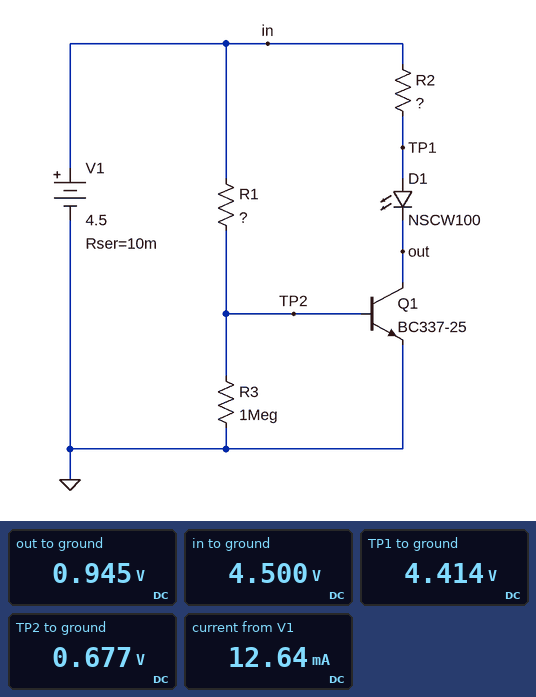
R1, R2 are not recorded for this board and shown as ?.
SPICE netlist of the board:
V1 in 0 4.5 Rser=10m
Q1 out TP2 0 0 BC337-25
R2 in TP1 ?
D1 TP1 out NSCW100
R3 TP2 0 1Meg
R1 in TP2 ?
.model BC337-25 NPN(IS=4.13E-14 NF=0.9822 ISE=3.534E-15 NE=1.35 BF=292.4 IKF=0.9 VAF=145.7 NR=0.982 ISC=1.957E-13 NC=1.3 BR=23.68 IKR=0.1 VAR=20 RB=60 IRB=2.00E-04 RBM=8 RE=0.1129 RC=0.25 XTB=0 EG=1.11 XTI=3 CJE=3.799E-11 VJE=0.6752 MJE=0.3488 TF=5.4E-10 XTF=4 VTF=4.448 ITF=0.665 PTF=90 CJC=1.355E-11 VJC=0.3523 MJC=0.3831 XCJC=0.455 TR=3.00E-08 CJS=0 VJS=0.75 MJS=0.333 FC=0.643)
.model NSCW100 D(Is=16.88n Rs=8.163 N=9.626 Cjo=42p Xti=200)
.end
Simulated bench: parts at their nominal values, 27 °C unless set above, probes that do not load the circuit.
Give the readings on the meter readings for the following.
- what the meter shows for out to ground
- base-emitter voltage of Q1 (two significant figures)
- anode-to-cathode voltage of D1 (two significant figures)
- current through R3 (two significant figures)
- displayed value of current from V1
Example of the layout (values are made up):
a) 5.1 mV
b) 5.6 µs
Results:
a) 0.945 V
b) 680 mV
c) 3.5 V
d) 680 nA
e) 12.64 mA
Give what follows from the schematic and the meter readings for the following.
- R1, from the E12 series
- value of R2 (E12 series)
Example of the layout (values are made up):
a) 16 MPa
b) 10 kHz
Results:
a) 82 kΩ
b) 6.8 Ω
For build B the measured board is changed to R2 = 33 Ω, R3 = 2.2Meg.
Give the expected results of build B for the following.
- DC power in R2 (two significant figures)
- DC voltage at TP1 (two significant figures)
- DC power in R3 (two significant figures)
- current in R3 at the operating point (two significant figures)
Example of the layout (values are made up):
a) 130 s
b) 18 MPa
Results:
a) 5.3 mW
b) 4.1 V
c) 210 nW
d) 310 nA
